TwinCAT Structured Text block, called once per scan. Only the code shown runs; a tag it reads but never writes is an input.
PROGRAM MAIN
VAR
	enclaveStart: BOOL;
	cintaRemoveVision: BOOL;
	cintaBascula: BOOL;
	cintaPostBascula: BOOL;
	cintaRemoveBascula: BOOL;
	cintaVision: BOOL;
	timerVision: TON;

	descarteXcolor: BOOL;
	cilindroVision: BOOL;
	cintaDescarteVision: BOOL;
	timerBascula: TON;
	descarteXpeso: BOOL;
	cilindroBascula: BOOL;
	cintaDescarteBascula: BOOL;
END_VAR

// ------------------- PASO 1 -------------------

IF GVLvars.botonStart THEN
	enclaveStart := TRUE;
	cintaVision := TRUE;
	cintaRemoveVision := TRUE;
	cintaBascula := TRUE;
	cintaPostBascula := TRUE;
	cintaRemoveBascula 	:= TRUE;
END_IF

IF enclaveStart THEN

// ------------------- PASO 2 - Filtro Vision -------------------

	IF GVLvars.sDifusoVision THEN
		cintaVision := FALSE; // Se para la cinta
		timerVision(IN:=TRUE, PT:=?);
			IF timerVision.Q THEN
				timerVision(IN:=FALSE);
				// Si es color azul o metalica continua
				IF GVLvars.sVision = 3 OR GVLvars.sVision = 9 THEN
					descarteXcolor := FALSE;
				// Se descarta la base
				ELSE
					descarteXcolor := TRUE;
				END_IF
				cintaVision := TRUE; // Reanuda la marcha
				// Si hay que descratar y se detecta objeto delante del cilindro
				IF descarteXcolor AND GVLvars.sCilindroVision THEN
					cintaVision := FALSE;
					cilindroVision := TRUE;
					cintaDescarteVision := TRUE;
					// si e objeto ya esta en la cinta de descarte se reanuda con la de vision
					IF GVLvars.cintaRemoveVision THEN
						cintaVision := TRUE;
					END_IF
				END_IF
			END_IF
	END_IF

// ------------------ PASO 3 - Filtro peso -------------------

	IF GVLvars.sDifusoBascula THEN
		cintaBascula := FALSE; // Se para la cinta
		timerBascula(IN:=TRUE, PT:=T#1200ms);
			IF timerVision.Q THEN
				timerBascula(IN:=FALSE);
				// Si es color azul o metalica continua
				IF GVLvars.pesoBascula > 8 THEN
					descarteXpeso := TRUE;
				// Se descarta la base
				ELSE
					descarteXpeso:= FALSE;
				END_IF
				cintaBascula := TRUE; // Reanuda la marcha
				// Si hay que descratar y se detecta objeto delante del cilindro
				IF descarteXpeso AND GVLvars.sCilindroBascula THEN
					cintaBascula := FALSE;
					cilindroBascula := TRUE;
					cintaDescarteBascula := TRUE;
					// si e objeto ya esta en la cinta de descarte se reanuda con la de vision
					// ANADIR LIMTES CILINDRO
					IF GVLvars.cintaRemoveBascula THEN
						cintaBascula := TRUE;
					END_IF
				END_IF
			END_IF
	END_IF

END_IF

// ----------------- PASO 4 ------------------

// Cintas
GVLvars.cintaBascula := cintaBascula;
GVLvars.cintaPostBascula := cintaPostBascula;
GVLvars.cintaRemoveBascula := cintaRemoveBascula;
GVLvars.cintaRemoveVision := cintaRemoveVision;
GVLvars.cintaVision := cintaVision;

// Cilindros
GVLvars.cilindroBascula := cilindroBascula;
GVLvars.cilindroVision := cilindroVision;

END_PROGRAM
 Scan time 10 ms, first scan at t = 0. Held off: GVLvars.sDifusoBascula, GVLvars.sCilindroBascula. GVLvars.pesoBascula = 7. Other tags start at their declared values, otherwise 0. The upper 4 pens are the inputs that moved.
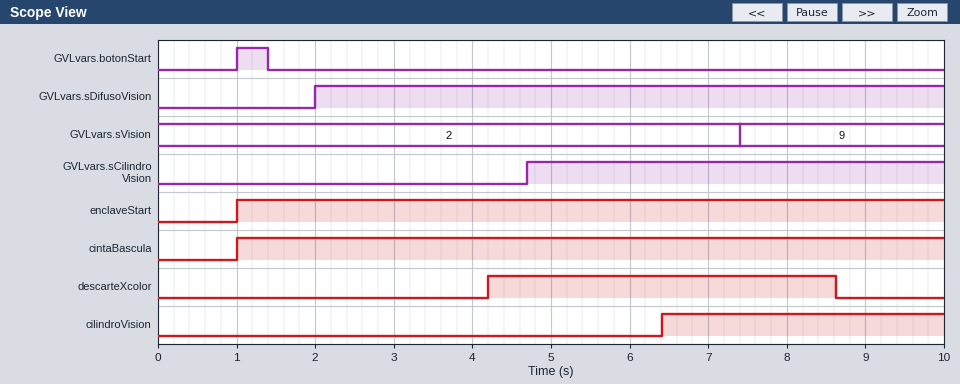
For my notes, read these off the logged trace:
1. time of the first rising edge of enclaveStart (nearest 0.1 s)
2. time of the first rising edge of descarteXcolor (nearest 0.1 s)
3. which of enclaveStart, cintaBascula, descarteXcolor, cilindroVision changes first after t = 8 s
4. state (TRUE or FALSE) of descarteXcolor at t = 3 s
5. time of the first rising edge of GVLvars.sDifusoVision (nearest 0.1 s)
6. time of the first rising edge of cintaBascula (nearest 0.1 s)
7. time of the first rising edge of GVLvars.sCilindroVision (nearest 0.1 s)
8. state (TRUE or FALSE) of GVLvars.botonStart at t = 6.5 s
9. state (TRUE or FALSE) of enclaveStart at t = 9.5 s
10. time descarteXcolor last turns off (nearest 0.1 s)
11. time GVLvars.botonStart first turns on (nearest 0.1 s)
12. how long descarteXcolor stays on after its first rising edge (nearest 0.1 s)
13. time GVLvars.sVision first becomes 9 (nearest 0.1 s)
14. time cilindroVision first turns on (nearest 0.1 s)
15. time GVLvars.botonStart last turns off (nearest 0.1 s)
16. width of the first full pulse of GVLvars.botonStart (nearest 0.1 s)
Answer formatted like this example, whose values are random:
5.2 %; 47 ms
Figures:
1.0 s; 4.2 s; descarteXcolor; FALSE; 2.0 s; 1.0 s; 4.7 s; FALSE; TRUE; 8.6 s; 1.0 s; 4.4 s; 7.4 s; 6.4 s; 1.4 s; 0.4 s
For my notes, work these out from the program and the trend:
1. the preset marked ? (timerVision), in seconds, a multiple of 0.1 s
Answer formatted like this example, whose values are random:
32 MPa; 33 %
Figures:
2.2 s
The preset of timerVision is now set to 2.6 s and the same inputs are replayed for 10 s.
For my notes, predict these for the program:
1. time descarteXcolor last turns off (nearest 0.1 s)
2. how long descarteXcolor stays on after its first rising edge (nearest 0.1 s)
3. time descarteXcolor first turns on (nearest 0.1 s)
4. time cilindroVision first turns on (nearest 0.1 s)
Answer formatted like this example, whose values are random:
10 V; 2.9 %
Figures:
9.8 s; 5.2 s; 4.6 s; 7.2 s
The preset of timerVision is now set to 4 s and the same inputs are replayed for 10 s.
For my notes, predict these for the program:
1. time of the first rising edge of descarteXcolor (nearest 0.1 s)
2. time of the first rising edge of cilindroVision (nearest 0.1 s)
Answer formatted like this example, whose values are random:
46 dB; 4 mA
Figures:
6.0 s; 6.0 s
